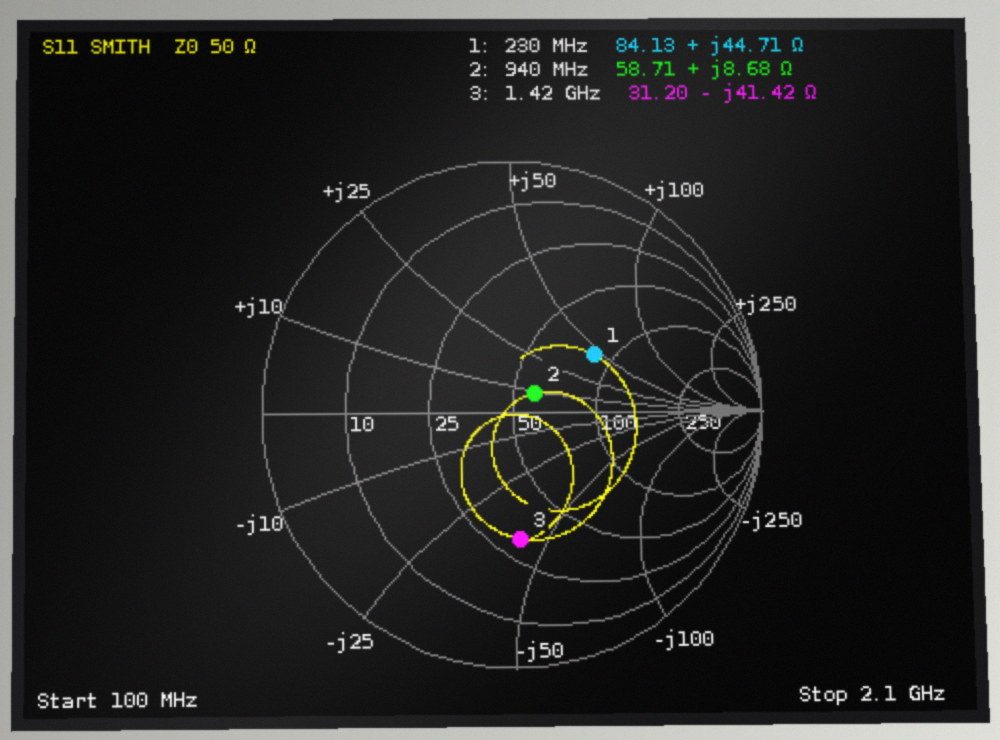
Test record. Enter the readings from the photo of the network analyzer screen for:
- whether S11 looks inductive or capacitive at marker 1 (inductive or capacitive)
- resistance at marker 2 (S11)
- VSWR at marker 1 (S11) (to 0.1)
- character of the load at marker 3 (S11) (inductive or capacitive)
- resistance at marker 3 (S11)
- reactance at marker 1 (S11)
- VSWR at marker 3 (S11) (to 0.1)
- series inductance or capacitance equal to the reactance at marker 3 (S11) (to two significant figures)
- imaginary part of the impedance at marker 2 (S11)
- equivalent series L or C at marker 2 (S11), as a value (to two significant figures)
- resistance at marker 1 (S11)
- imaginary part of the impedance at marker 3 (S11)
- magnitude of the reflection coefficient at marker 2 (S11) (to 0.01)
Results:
inductive
58.71 Ω
2.3
capacitive
31.20 Ω
+44.71 Ω
3.0
2.7 pF
+8.68 Ω
1.5 nH
84.13 Ω
-41.42 Ω
0.11
